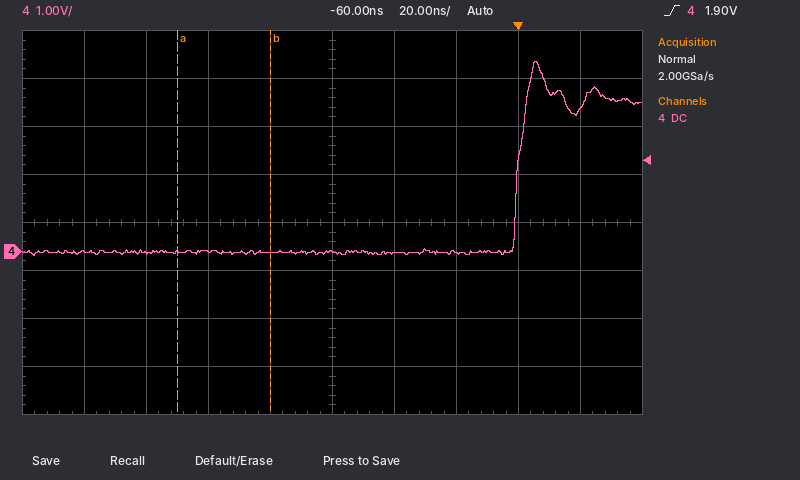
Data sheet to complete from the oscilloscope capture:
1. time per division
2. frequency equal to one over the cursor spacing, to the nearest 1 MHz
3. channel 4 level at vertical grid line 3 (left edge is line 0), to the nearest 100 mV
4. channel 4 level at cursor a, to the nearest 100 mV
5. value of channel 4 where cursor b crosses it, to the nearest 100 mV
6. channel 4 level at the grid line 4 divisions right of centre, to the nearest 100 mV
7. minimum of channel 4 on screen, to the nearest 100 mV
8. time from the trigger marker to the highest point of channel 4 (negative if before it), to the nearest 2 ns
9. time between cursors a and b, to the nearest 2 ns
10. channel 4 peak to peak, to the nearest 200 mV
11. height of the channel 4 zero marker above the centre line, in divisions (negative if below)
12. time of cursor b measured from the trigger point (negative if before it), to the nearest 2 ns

20 ns
33 MHz
0.0 V
0.0 V
0.0 V
3.0 V
-100 mV
+6 ns
30 ns
4.0 V
-0.6 div
-80 ns
